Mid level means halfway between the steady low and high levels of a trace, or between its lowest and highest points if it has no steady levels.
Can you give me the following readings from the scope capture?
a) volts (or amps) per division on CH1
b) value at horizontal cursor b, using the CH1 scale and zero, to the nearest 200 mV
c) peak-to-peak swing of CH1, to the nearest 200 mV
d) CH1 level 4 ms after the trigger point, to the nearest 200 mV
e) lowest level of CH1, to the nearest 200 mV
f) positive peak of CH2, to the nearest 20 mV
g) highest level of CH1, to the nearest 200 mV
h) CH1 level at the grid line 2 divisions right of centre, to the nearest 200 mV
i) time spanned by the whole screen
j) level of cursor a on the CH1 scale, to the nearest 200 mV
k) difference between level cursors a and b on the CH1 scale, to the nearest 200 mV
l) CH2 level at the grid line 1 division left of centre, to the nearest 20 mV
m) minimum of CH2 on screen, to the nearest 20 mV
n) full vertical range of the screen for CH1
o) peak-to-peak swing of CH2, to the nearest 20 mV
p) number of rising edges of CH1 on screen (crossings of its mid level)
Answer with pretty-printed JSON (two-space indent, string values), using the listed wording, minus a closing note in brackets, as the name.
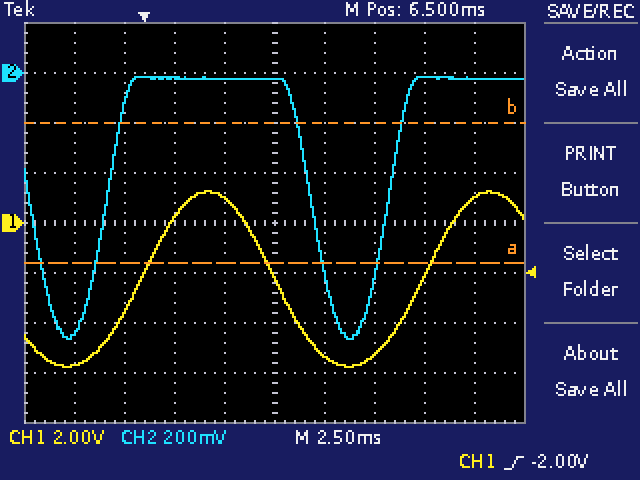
{
  "volts (or amps) per division on CH1": "2 V",
  "value at horizontal cursor b, using the CH1 scale and zero, to the nearest 200 mV": "4.0 V",
  "peak-to-peak swing of CH1, to the nearest 200 mV": "7.0 V",
  "CH1 level 4 ms after the trigger point, to the nearest 200 mV": "1.0 V",
  "lowest level of CH1, to the nearest 200 mV": "-5.8 V",
  "positive peak of CH2, to the nearest 20 mV": "-20 mV",
  "highest level of CH1, to the nearest 200 mV": "1.2 V",
  "CH1 level at the grid line 2 divisions right of centre, to the nearest 200 mV": "-5.2 V",
  "time spanned by the whole screen": "25 ms",
  "level of cursor a on the CH1 scale, to the nearest 200 mV": "-1.6 V",
  "difference between level cursors a and b on the CH1 scale, to the nearest 200 mV": "5.6 V",
  "CH2 level at the grid line 1 division left of centre, to the nearest 20 mV": "-20 mV",
  "minimum of CH2 on screen, to the nearest 20 mV": "-1.06 V",
  "full vertical range of the screen for CH1": "16 V",
  "peak-to-peak swing of CH2, to the nearest 20 mV": "1.04 V",
  "number of rising edges of CH1 on screen": "2"
}
